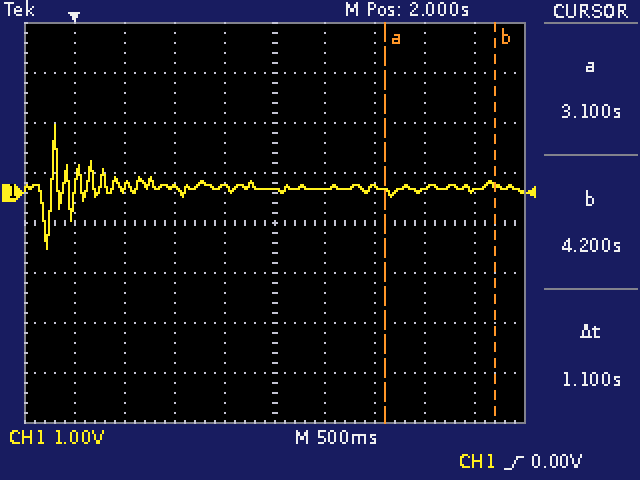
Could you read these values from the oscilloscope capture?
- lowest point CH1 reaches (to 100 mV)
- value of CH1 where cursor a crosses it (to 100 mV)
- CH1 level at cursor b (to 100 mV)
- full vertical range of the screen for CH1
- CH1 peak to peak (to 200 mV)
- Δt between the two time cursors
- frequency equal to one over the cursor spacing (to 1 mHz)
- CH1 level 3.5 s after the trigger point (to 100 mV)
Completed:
-1.1 V
0.0 V
200 mV
8 V
2.4 V
1.1 s
909 mHz
100 mV
